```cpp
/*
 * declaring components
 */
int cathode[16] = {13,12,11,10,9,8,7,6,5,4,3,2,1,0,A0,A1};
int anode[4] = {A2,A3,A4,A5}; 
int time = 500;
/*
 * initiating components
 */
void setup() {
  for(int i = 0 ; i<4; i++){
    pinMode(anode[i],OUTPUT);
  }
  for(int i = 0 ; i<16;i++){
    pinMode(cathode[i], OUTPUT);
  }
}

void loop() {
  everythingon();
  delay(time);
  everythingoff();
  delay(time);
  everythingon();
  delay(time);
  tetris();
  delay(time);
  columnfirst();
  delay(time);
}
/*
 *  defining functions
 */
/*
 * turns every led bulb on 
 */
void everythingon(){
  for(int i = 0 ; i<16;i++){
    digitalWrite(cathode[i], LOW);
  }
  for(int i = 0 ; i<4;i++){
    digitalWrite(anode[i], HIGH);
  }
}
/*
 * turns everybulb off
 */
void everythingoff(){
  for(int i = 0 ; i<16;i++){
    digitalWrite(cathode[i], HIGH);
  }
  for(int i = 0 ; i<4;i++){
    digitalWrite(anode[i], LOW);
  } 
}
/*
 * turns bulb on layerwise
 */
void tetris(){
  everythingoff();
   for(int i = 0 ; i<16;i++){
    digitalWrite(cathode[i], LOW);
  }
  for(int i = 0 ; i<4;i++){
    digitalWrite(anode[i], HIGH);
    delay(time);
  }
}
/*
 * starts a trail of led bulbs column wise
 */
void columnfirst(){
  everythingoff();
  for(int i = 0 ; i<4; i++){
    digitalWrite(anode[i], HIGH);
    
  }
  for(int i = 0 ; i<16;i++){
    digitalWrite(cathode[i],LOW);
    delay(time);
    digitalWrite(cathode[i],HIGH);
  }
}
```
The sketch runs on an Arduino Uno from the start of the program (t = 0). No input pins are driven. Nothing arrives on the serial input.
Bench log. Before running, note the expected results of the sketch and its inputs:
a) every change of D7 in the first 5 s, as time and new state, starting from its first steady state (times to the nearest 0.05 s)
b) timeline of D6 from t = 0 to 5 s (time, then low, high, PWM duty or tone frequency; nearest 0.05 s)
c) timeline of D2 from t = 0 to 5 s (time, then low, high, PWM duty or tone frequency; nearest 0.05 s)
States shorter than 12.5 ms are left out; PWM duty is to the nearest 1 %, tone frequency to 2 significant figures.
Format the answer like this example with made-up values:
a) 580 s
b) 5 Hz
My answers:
a) 0 s low; 0.5 s high; 1 s low; 4 s high
b) 0 s low; 0.5 s high; 1 s low; 4 s high
c) 0 s low; 0.5 s high; 1 s low; 4 s high
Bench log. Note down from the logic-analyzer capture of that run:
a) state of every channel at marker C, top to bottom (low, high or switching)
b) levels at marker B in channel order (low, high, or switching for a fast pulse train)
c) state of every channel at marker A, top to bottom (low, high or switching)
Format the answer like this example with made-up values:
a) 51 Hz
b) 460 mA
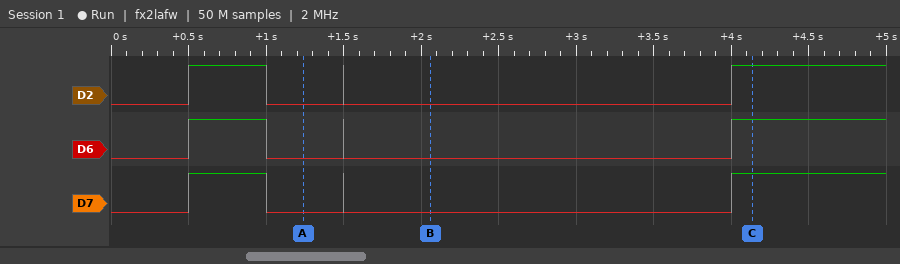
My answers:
a) D2 high, D6 high, D7 high
b) D2 low, D6 low, D7 low
c) D2 low, D6 low, D7 low
